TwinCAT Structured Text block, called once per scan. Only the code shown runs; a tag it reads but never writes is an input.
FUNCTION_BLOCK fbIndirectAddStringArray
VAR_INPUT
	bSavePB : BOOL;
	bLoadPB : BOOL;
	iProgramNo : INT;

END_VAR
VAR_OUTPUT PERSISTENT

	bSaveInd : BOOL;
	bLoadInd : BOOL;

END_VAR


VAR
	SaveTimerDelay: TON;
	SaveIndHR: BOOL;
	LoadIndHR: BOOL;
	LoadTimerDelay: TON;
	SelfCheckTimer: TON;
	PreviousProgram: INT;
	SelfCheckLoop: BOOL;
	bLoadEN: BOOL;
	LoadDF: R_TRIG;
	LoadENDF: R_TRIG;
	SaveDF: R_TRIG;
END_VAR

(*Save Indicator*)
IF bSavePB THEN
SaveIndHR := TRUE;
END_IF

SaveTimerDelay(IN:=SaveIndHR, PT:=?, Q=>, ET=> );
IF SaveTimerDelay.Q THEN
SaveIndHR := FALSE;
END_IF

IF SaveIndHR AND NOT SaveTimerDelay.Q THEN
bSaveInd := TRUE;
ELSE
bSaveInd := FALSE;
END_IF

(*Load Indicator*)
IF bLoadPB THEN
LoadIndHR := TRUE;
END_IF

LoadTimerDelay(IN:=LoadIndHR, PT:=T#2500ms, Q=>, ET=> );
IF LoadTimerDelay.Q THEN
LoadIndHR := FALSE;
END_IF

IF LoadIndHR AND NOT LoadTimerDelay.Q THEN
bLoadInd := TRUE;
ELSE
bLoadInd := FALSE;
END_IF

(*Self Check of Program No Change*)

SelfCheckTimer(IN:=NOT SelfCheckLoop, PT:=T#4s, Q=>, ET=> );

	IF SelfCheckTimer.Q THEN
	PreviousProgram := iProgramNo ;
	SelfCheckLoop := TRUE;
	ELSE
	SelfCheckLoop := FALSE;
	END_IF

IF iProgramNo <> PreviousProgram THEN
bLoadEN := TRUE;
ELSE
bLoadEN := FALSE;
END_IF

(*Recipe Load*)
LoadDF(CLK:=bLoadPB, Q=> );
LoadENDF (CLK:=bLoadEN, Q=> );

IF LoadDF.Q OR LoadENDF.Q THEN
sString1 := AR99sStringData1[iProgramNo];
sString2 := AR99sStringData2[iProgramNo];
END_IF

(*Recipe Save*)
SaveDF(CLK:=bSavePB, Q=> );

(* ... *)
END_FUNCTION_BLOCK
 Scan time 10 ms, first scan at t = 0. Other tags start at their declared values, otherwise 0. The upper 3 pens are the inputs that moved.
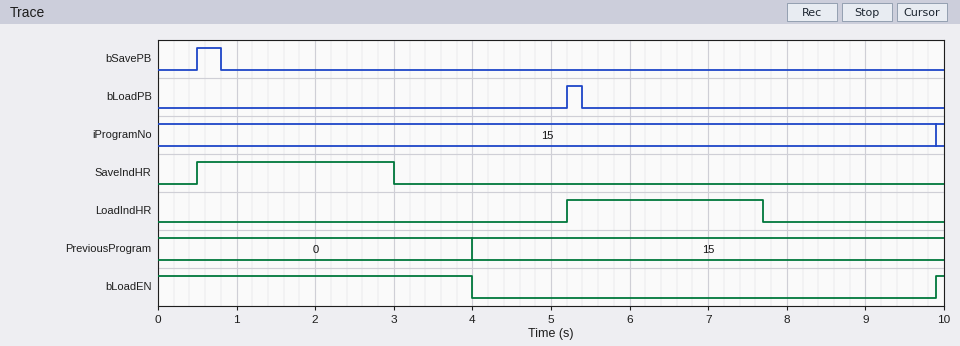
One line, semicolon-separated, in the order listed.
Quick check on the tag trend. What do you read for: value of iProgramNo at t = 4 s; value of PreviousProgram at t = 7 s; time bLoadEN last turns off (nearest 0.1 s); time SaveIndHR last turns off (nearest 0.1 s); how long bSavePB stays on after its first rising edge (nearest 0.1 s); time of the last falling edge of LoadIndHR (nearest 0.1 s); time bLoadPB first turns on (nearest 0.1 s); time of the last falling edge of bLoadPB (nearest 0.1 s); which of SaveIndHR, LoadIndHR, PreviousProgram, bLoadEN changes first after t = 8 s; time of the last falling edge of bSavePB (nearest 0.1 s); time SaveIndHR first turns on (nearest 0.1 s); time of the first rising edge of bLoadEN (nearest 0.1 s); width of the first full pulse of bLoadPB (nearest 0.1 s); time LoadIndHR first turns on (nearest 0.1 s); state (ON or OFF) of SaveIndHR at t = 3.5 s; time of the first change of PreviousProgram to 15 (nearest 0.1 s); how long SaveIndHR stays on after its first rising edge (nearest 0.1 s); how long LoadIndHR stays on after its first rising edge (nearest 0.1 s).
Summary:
15; 15; 4.0 s; 3.0 s; 0.3 s; 7.7 s; 5.2 s; 5.4 s; bLoadEN; 0.8 s; 0.5 s; 9.9 s; 0.2 s; 5.2 s; OFF; 4.0 s; 2.5 s; 2.5 s
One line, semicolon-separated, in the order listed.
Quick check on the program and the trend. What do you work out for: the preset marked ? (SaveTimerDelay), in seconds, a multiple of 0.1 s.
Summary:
2.5 s
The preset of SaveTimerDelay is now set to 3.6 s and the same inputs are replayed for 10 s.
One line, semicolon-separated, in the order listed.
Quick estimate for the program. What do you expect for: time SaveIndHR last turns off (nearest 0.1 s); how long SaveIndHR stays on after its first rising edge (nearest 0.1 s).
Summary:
4.1 s; 3.6 s
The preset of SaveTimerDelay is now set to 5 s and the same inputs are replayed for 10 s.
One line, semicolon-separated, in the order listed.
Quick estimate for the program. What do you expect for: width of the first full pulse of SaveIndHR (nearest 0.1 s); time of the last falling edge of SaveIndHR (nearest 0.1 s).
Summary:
5.0 s; 5.5 s
